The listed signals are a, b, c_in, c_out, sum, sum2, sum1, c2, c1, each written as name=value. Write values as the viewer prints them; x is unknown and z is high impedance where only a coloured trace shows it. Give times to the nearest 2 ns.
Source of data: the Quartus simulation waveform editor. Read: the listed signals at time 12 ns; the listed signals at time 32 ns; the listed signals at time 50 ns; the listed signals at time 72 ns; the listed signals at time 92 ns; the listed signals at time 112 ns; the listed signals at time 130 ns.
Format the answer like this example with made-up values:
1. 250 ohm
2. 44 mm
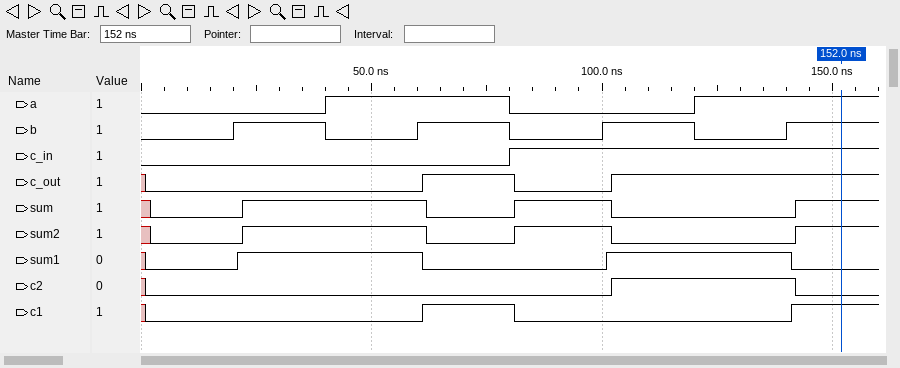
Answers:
1. a=0, b=0, c_in=0, c_out=0, sum=0, sum2=0, sum1=0, c2=0, c1=0
2. a=0, b=1, c_in=0, c_out=0, sum=1, sum2=1, sum1=1, c2=0, c1=0
3. a=1, b=0, c_in=0, c_out=0, sum=1, sum2=1, sum1=1, c2=0, c1=0
4. a=1, b=1, c_in=0, c_out=1, sum=0, sum2=0, sum1=0, c2=0, c1=1
5. a=0, b=0, c_in=1, c_out=0, sum=1, sum2=1, sum1=0, c2=0, c1=0
6. a=0, b=1, c_in=1, c_out=1, sum=0, sum2=0, sum1=1, c2=1, c1=0
7. a=1, b=0, c_in=1, c_out=1, sum=0, sum2=0, sum1=1, c2=1, c1=0
